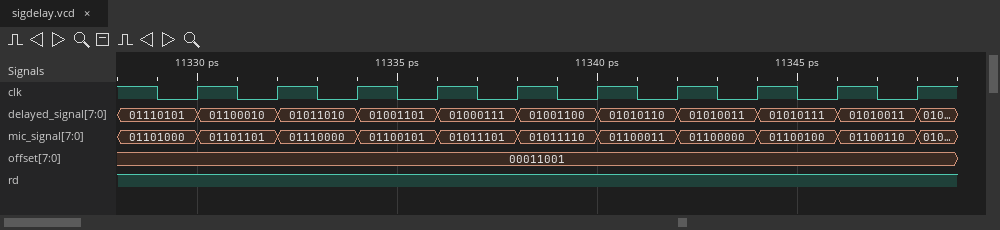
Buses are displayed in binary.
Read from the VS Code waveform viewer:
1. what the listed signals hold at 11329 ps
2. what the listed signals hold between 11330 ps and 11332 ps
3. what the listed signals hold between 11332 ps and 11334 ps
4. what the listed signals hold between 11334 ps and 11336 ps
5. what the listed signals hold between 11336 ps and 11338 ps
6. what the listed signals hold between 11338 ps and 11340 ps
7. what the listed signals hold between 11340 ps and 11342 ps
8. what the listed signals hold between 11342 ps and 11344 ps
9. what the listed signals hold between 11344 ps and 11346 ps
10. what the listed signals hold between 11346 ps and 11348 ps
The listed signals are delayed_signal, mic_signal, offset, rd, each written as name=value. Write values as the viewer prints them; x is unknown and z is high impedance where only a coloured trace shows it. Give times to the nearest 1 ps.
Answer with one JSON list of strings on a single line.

["delayed_signal=01110101, mic_signal=01101000, offset=00011001, rd=1", "delayed_signal=01100010, mic_signal=01101101, offset=00011001, rd=1", "delayed_signal=01011010, mic_signal=01110000, offset=00011001, rd=1", "delayed_signal=01001101, mic_signal=01100101, offset=00011001, rd=1", "delayed_signal=01000111, mic_signal=01011101, offset=00011001, rd=1", "delayed_signal=01001100, mic_signal=01011110, offset=00011001, rd=1", "delayed_signal=01010110, mic_signal=01100011, offset=00011001, rd=1", "delayed_signal=01010011, mic_signal=01100000, offset=00011001, rd=1", "delayed_signal=01010111, mic_signal=01100100, offset=00011001, rd=1", "delayed_signal=01010011, mic_signal=01100110, offset=00011001, rd=1"]
